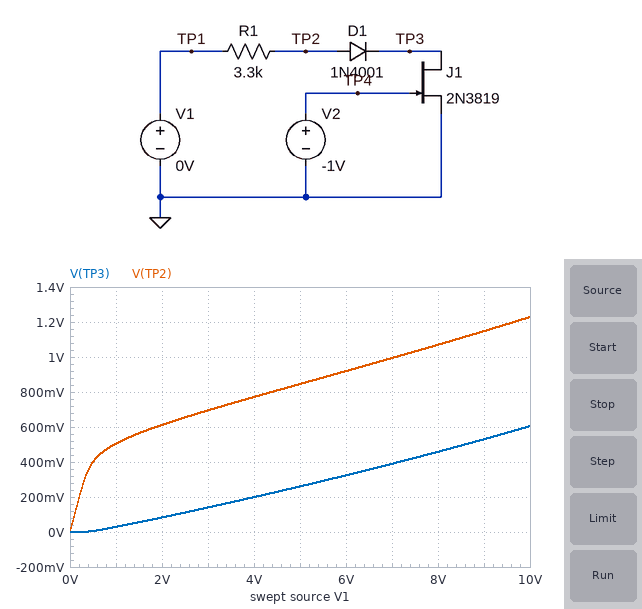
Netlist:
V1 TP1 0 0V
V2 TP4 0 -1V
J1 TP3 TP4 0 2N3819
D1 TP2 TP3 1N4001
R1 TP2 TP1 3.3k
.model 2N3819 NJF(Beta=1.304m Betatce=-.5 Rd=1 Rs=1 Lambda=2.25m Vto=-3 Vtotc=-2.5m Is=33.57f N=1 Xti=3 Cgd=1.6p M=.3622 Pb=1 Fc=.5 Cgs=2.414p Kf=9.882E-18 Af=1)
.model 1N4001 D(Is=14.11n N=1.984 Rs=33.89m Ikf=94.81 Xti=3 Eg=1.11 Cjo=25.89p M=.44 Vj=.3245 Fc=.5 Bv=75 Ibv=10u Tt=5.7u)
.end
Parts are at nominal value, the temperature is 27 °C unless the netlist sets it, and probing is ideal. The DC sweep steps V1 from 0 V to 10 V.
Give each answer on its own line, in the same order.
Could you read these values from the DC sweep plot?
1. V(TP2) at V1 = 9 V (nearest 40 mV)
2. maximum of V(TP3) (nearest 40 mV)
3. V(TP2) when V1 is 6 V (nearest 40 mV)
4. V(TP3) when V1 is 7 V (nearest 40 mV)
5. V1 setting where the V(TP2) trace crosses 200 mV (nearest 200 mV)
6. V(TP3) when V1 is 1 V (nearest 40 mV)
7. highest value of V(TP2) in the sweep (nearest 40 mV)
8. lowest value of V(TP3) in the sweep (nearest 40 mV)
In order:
1.16 V
600 mV
920 mV
400 mV
200 mV
40 mV
1.24 V
0 V
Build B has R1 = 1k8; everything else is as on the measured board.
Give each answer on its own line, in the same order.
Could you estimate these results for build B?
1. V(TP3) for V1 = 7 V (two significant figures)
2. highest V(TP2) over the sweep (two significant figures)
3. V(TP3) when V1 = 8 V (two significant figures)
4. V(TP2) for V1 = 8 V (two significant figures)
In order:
740 mV
1.9 V
890 mV
1.5 V
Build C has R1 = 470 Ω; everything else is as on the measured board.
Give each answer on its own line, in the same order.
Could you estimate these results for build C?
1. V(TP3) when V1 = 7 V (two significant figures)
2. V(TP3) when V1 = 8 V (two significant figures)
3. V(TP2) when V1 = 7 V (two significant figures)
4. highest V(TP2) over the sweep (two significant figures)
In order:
3.9 V
4.9 V
4.5 V
7.5 V
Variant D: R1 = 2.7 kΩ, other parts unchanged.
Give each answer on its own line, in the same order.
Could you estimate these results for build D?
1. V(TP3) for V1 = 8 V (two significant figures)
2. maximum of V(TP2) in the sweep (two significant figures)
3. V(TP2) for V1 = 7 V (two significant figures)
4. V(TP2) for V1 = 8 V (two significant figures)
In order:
570 mV
1.4 V
1.1 V
1.2 V
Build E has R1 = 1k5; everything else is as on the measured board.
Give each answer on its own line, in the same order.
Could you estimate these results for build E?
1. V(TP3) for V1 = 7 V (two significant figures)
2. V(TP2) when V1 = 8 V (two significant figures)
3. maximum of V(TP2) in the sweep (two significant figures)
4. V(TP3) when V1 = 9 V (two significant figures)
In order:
910 mV
1.8 V
2.4 V
1.4 V
